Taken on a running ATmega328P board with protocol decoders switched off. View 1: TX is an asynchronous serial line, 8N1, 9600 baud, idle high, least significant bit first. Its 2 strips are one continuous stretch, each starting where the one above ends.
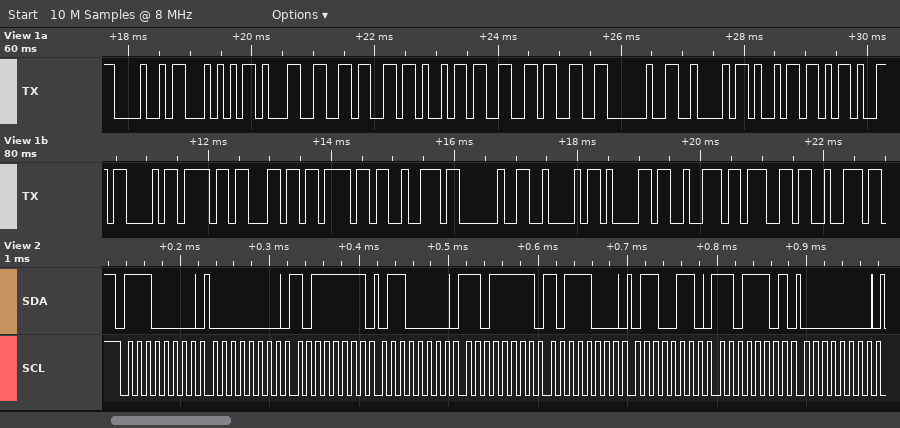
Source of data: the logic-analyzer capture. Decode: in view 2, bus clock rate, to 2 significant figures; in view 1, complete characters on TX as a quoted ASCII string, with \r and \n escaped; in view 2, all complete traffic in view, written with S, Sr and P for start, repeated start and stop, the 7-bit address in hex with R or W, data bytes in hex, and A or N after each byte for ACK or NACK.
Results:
100 kHz
"HT16K33 Bi-Color Bargr"
S 70W A 00 A BF A 60 A DF A B8 A 66 A DD A 00 A
